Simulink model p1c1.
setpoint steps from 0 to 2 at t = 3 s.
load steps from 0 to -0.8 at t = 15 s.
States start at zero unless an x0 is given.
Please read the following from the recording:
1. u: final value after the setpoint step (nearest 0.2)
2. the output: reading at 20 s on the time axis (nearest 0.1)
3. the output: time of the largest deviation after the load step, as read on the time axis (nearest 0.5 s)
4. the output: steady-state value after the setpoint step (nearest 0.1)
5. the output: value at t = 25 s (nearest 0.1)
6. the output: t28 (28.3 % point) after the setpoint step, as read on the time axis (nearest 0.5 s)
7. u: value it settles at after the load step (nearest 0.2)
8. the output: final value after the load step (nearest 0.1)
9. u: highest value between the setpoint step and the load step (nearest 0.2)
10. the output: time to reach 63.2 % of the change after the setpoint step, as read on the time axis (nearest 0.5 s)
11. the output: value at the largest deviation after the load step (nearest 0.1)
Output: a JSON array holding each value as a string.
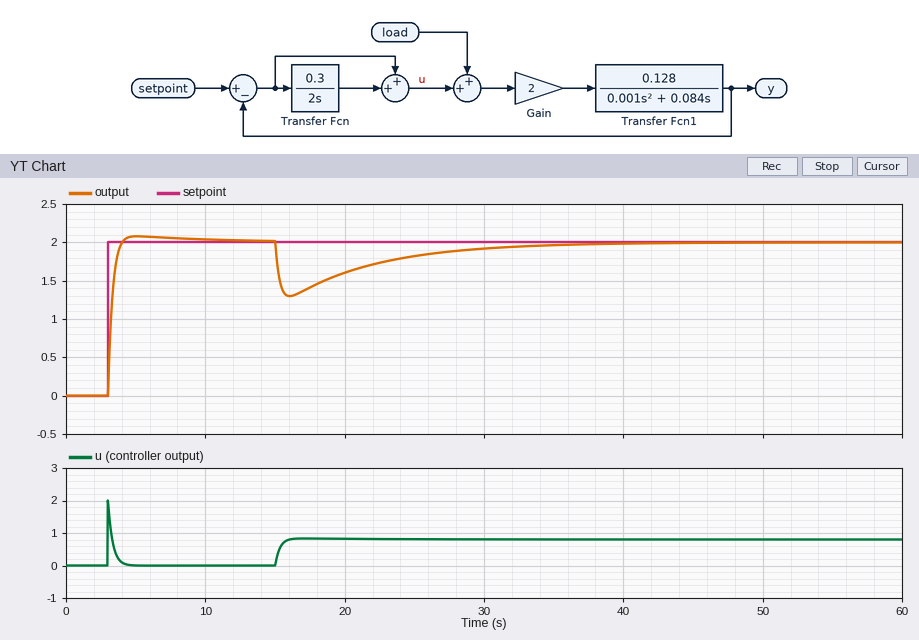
["0.0", "1.6", "16.0 s", "2.0", "1.8", "3.0 s", "0.8", "2.0", "2.0", "3.5 s", "1.3"]
